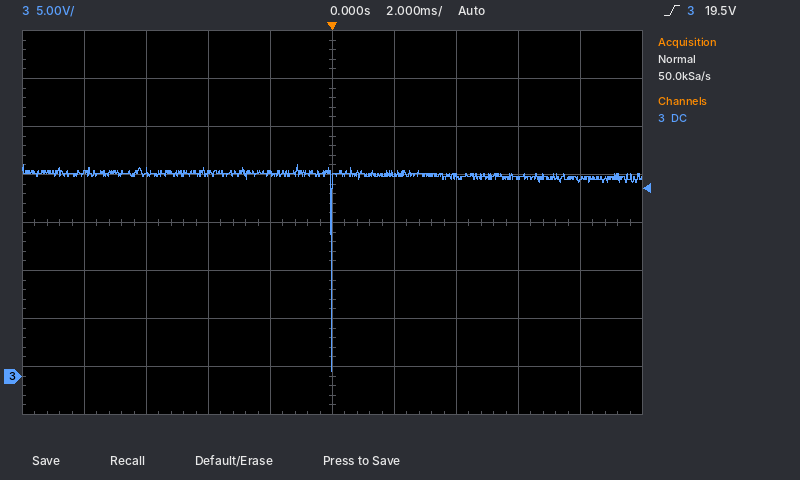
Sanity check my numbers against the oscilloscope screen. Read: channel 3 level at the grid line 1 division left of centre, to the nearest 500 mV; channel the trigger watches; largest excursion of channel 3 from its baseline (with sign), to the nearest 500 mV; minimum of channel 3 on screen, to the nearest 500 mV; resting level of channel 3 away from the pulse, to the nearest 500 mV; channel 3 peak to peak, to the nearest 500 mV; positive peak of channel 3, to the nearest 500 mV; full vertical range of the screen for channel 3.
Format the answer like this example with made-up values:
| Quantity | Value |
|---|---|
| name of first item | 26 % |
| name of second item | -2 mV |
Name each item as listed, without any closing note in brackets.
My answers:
| Quantity | Value |
|---|---|
| channel 3 level at the grid line 1 division left of centre, to the nearest 500 mV | 21.0 V |
| channel the trigger watches | channel 3 |
| largest excursion of channel 3 from its baseline (with sign), to the nearest 500 mV | -20.5 V |
| minimum of channel 3 on screen, to the nearest 500 mV | 500 mV |
| resting level of channel 3 away from the pulse, to the nearest 500 mV | 21.0 V |
| channel 3 peak to peak, to the nearest 500 mV | 21.5 V |
| positive peak of channel 3, to the nearest 500 mV | 22.0 V |
| full vertical range of the screen for channel 3 | 40 V |
